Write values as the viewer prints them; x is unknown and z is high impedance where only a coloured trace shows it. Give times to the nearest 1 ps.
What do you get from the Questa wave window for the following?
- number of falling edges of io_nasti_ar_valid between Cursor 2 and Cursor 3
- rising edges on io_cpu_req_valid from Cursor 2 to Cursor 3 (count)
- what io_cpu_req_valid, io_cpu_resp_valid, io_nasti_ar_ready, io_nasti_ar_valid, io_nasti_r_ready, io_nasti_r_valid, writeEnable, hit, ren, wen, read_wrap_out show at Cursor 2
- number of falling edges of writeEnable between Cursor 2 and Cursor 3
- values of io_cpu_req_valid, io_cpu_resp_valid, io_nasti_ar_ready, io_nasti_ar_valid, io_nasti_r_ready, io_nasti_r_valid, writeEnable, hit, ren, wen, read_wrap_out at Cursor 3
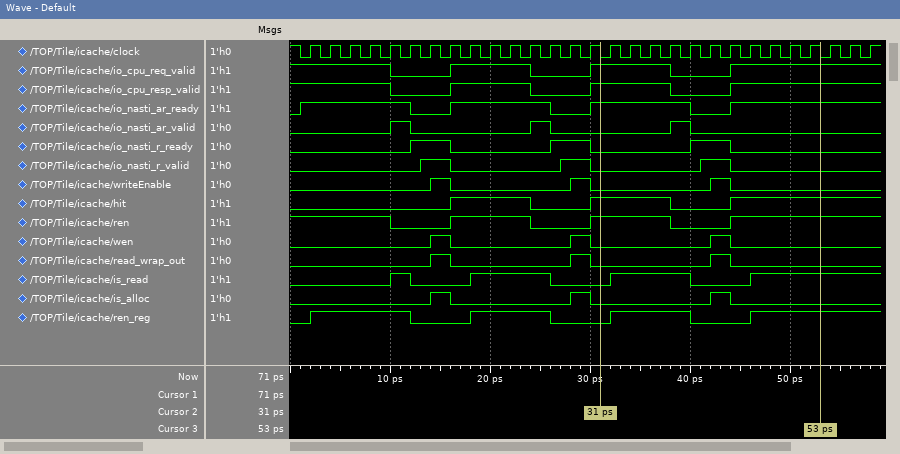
1
1
io_cpu_req_valid=1, io_cpu_resp_valid=1, io_nasti_ar_ready=1, io_nasti_ar_valid=0, io_nasti_r_ready=0, io_nasti_r_valid=0, writeEnable=0, hit=1, ren=1, wen=0, read_wrap_out=0
1
io_cpu_req_valid=1, io_cpu_resp_valid=1, io_nasti_ar_ready=1, io_nasti_ar_valid=0, io_nasti_r_ready=0, io_nasti_r_valid=0, writeEnable=0, hit=1, ren=1, wen=0, read_wrap_out=0
